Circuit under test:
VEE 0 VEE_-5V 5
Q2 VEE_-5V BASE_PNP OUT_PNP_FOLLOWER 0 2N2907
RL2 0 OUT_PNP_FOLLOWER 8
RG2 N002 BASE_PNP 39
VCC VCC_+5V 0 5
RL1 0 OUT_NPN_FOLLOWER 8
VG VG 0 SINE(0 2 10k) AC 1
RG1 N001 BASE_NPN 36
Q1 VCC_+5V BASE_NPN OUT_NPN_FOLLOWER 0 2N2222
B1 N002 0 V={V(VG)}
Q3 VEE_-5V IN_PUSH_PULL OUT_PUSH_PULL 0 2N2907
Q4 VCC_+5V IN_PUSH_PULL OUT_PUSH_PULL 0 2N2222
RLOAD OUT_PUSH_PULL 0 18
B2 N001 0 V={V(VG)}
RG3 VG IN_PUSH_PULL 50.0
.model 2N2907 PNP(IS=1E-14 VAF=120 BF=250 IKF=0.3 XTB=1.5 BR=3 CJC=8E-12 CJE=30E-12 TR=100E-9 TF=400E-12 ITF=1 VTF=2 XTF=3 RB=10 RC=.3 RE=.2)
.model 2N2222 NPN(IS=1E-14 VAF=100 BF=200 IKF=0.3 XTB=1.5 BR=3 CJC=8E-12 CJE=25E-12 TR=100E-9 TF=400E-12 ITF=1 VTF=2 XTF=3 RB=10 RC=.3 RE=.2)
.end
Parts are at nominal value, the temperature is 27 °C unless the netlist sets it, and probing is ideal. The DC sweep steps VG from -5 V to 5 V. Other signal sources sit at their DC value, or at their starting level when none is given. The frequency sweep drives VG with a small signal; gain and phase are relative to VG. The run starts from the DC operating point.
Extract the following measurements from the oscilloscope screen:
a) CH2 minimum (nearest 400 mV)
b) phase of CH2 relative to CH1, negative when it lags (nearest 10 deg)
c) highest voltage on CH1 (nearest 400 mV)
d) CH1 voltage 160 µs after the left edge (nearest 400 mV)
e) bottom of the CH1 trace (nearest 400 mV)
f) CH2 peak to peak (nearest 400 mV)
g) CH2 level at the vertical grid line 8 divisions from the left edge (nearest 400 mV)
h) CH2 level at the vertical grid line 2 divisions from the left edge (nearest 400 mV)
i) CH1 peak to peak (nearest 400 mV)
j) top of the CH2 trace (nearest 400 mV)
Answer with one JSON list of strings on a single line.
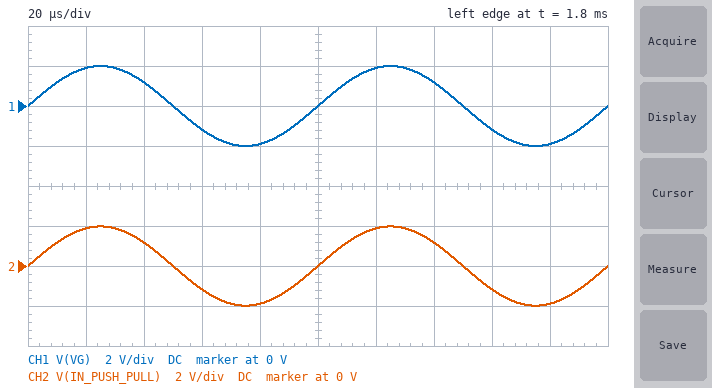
["-2.0 V", "0 deg", "2.0 V", "-1.2 V", "-2.0 V", "4.0 V", "-1.2 V", "1.2 V", "4.0 V", "2.0 V"]
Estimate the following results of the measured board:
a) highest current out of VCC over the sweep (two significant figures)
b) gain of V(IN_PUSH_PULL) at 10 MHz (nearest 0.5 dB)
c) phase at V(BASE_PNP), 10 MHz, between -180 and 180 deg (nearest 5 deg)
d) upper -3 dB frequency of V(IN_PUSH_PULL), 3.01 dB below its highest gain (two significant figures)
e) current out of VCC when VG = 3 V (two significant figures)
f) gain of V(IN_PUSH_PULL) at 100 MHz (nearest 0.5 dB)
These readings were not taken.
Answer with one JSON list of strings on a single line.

["690 mA", "-0.5 dB", "-5 deg", "40 MHz", "370 mA", "-7.0 dB"]
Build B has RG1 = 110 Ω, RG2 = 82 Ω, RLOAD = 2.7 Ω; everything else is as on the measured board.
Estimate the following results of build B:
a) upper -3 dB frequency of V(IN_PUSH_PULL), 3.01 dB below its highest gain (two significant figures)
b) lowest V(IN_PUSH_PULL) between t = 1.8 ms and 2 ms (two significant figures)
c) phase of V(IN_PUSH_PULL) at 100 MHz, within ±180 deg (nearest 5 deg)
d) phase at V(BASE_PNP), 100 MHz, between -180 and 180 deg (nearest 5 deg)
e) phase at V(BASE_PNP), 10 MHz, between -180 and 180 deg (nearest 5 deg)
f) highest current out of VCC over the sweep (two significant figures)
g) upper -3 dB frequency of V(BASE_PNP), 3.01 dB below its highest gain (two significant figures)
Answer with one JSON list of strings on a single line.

["45 MHz", "-1.9 V", "-50 deg", "-45 deg", "-10 deg", "1.4 A", "49 MHz"]
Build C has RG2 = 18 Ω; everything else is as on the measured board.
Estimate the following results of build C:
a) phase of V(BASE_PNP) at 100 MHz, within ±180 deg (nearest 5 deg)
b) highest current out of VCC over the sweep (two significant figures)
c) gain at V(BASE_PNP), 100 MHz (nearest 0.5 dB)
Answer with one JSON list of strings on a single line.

["-15 deg", "690 mA", "-1.5 dB"]
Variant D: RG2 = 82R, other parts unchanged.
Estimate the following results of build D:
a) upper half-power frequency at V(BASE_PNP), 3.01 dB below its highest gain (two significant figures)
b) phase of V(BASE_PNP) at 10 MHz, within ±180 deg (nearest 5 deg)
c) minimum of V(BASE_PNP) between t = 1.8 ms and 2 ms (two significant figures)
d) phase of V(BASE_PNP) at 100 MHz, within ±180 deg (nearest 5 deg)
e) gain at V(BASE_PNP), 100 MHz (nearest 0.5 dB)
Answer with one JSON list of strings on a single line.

["49 MHz", "-10 deg", "-1.9 V", "-45 deg", "-7.0 dB"]
